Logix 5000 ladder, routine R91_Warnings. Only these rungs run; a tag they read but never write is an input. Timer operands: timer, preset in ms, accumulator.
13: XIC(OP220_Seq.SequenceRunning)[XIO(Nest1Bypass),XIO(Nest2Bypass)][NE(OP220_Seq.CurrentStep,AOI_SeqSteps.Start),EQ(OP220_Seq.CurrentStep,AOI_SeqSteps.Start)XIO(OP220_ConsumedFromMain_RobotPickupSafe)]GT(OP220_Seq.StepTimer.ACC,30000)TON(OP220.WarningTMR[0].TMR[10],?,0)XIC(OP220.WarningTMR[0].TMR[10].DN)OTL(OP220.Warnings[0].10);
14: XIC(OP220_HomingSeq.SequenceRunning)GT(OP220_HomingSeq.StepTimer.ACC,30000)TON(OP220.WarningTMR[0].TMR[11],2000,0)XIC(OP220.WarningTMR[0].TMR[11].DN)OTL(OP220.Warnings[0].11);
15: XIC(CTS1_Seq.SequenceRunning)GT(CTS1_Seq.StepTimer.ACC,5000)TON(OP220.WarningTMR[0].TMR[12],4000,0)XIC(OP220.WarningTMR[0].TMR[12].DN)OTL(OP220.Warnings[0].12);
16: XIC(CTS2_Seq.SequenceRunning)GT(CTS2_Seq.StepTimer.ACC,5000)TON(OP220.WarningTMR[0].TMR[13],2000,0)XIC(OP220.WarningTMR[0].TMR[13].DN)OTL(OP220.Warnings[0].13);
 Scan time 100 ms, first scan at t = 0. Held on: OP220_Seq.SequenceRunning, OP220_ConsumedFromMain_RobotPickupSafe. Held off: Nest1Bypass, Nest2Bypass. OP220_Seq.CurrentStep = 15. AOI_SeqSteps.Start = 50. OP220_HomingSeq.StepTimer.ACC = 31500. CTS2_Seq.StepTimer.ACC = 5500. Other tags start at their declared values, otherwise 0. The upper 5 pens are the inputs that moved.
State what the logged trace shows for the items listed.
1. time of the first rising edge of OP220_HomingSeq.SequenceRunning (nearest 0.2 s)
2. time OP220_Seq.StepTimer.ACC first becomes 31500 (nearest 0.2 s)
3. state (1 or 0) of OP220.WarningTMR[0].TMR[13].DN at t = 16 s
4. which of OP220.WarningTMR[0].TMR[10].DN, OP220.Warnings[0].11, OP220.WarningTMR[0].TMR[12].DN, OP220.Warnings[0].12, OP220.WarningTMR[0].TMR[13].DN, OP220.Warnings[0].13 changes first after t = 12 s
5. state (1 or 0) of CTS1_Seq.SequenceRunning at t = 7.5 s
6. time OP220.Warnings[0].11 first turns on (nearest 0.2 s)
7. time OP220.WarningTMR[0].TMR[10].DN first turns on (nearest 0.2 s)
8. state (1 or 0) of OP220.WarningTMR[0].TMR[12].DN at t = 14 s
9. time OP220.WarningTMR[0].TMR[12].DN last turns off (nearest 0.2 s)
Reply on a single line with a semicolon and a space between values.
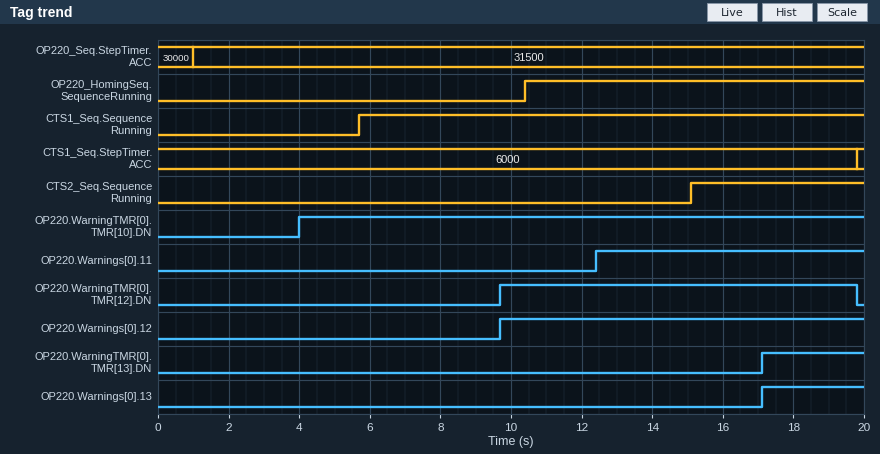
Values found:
10.4 s; 1.0 s; 0; OP220.Warnings[0].11; 1; 12.4 s; 4.0 s; 1; 19.8 s
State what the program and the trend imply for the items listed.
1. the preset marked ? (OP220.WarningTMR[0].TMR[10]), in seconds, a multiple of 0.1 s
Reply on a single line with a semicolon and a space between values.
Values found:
3.0 s
